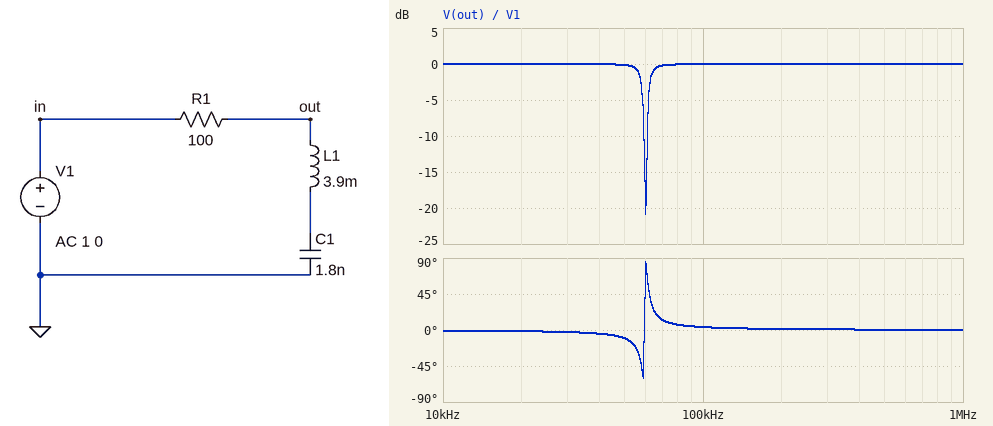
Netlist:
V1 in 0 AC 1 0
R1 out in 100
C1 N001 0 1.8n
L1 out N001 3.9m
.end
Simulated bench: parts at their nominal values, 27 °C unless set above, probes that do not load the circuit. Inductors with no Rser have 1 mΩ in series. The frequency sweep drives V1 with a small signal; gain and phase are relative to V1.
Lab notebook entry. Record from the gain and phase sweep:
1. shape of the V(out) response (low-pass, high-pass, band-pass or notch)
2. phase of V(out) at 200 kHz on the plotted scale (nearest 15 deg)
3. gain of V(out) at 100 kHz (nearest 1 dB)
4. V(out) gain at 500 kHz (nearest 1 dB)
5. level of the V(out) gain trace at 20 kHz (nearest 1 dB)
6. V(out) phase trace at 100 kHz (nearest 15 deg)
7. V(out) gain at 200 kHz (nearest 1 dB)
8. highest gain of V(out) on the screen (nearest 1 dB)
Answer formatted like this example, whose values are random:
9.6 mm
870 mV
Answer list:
notch
0 deg
0 dB
0 dB
0 dB
0 deg
0 dB
0 dB
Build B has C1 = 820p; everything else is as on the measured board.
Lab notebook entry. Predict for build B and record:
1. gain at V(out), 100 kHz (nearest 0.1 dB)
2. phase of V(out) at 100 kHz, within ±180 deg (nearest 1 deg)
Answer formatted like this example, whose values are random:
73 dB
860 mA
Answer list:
-0.2 dB
11 deg
